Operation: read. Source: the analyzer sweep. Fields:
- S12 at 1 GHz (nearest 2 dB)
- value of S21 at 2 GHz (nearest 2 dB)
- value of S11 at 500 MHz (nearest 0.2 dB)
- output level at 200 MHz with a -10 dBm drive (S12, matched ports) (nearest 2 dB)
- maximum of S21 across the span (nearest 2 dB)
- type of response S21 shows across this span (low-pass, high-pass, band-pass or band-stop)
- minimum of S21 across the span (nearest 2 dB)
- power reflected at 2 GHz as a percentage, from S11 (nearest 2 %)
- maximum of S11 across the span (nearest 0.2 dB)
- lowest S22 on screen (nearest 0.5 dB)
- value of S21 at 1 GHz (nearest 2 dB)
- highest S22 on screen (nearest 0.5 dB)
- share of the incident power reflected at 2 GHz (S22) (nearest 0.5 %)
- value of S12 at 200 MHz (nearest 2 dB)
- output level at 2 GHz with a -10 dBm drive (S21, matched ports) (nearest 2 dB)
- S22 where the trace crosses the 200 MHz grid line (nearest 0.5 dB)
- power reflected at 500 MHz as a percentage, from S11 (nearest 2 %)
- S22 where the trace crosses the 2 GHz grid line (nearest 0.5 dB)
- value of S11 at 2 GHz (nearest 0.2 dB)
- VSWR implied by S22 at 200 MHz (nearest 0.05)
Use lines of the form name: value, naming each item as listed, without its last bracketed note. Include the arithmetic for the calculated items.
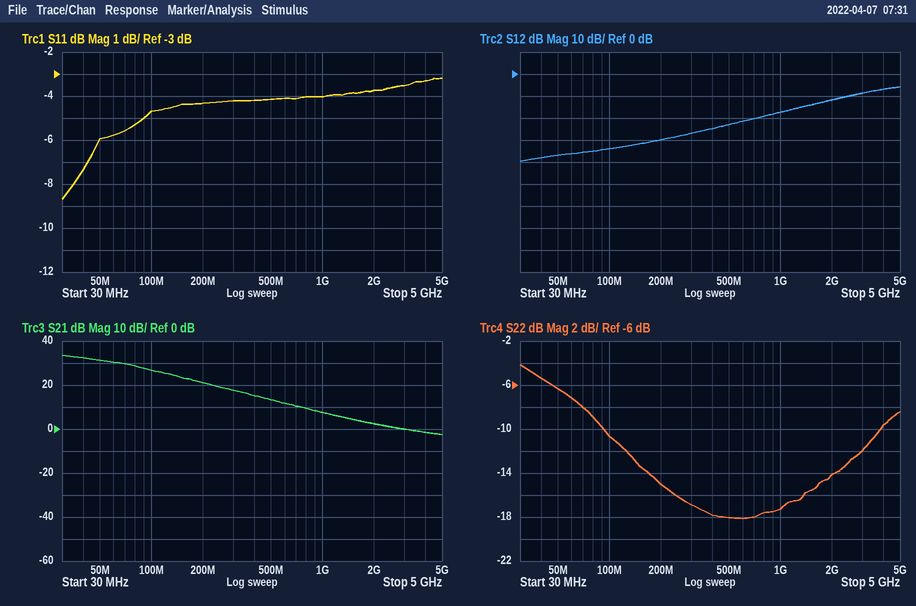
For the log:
S12 at 1 GHz: -18 dB
value of S21 at 2 GHz: 2 dB
value of S11 at 500 MHz: -4.2 dB
output level at 200 MHz with a -10 dBm drive (S12, matched ports): -10 dBm + (-30 dB) = -40 dBm
maximum of S21 across the span: 34 dB
type of response S21 shows across this span: low-pass
minimum of S21 across the span: -2 dB
power reflected at 2 GHz as a percentage, from S11: 10^(-3.8/10) ≈ 42 %
maximum of S11 across the span: -3.2 dB
lowest S22 on screen: -18.0 dB
value of S21 at 1 GHz: 8 dB
highest S22 on screen: -4.0 dB
share of the incident power reflected at 2 GHz (S22): 10^(-14/10) ≈ 4.0 %
value of S12 at 200 MHz: -30 dB
output level at 2 GHz with a -10 dBm drive (S21, matched ports): -10 dBm + (2 dB) = -8 dBm
S22 where the trace crosses the 200 MHz grid line: -15.0 dB
power reflected at 500 MHz as a percentage, from S11: 10^(-4.2/10) ≈ 38 %
S22 where the trace crosses the 2 GHz grid line: -14.0 dB
value of S11 at 2 GHz: -3.8 dB
VSWR implied by S22 at 200 MHz: |Γ| = 10^(-15/20) = 0.1778; VSWR = (1 + 0.1778)/(1 − 0.1778) ≈ 1.43, so 1.45 to the nearest 0.05
